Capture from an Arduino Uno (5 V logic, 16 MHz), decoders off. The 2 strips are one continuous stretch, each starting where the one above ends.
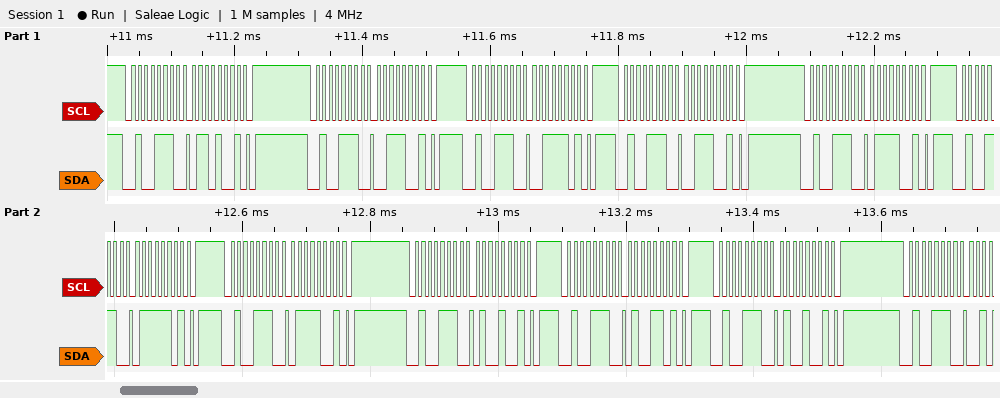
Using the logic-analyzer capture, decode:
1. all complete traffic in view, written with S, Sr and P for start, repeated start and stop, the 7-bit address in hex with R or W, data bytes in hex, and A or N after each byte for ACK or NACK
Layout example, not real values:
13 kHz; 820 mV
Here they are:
S 27W A 69 A P S 27W A 39 A P S 27W A 3D A P S 27W A 39 A P S 27W A 79 A P S 27W A 7D A P S 27W A 79 A P S 27W A 49 A P S 27W A 4D A P S 27W A 49 A P S 27W A
